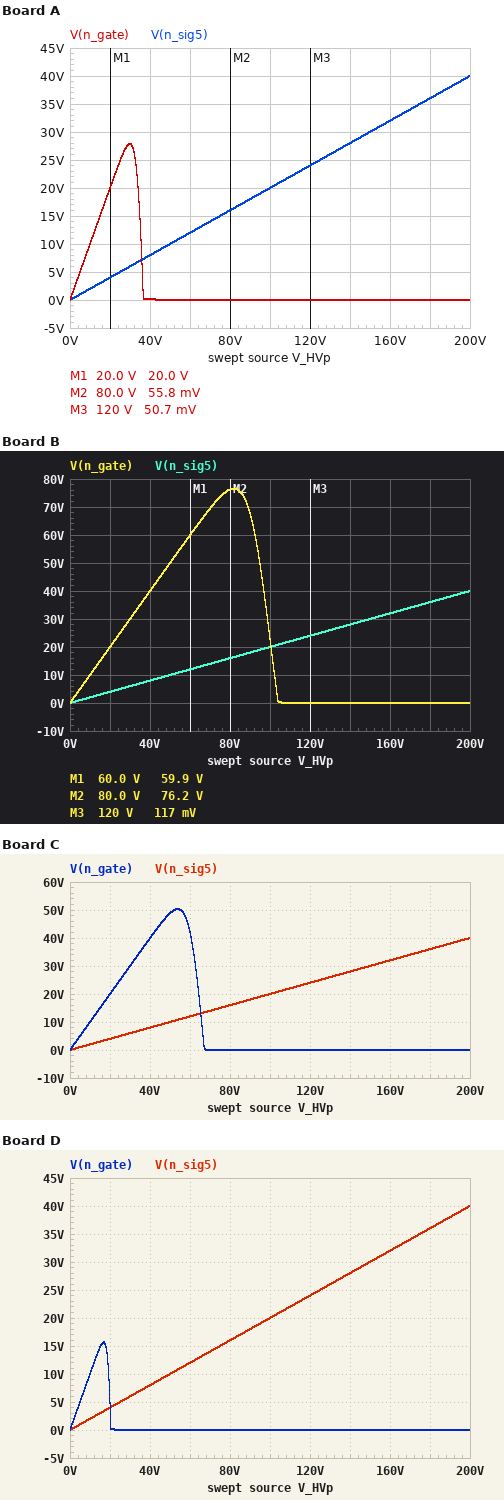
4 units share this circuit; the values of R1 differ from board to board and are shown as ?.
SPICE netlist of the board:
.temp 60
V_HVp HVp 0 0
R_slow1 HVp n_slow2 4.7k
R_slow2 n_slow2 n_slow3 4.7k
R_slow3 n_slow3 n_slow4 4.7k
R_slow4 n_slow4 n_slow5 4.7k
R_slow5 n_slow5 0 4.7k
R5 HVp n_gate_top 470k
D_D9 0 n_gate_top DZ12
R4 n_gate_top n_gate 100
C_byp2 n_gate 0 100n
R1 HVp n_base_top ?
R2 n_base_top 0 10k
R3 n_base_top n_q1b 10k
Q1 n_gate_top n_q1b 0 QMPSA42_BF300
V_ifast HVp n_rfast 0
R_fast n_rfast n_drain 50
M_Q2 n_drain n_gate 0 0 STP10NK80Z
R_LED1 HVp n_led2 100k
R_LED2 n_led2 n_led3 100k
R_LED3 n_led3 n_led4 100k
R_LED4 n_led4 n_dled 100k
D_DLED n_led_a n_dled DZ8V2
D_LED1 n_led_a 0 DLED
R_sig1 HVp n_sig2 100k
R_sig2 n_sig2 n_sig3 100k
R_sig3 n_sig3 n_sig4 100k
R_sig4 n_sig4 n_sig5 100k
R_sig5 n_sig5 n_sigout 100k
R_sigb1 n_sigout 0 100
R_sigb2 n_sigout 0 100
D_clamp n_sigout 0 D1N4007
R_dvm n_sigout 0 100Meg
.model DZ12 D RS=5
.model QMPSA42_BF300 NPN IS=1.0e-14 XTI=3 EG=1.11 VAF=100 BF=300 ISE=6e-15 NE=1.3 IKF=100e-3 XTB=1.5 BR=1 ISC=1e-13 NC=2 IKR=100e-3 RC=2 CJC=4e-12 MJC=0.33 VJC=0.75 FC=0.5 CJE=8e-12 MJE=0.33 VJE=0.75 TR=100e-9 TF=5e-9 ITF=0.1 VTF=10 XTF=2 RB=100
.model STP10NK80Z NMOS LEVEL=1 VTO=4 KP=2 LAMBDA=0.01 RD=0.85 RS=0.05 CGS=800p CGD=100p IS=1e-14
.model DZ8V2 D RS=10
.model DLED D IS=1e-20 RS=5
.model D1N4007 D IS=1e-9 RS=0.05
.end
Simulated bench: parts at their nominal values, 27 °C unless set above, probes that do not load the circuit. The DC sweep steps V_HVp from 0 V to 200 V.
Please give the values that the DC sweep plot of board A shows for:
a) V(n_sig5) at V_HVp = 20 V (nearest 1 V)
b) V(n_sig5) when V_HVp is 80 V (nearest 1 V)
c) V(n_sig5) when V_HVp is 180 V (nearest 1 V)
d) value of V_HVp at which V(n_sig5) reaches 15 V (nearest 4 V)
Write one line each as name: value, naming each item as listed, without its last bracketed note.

V(n_sig5) at V_HVp = 20 V: 4 V
V(n_sig5) when V_HVp is 80 V: 16 V
V(n_sig5) when V_HVp is 180 V: 36 V
value of V_HVp at which V(n_sig5) reaches 15 V: 76 V
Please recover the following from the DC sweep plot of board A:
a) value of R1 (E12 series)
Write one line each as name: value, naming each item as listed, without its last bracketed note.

value of R1: 680 kΩ
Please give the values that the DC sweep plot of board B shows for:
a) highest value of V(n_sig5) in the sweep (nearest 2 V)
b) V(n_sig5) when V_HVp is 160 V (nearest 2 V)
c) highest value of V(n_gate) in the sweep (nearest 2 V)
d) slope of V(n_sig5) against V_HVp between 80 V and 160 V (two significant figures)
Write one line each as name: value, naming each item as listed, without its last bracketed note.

highest value of V(n_sig5) in the sweep: 40 V
V(n_sig5) when V_HVp is 160 V: 32 V
highest value of V(n_gate) in the sweep: 76 V
slope of V(n_sig5) against V_HVp between 80 V and 160 V: 0.20 V/V
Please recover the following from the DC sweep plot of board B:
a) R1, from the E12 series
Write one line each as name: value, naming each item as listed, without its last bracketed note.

R1, from the E12 series: 1.8 MΩ
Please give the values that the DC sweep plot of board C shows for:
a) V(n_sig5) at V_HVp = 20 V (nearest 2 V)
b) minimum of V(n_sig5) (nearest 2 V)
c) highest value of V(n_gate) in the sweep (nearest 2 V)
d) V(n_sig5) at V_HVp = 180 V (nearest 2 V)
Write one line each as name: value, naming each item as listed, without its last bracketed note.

V(n_sig5) at V_HVp = 20 V: 4 V
minimum of V(n_sig5): 0 V
highest value of V(n_gate) in the sweep: 50 V
V(n_sig5) at V_HVp = 180 V: 36 V
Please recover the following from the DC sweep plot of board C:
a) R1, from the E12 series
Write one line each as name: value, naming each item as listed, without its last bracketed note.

R1, from the E12 series: 1.2 MΩ
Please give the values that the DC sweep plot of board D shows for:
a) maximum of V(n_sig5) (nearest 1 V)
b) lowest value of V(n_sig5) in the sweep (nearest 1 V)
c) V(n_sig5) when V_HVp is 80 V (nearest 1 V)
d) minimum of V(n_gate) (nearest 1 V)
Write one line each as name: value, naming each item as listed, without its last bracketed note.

maximum of V(n_sig5): 40 V
lowest value of V(n_sig5) in the sweep: 0 V
V(n_sig5) when V_HVp is 80 V: 16 V
minimum of V(n_gate): 0 V
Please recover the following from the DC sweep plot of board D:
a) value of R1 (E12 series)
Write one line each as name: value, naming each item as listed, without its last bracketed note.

value of R1: 390 kΩ
